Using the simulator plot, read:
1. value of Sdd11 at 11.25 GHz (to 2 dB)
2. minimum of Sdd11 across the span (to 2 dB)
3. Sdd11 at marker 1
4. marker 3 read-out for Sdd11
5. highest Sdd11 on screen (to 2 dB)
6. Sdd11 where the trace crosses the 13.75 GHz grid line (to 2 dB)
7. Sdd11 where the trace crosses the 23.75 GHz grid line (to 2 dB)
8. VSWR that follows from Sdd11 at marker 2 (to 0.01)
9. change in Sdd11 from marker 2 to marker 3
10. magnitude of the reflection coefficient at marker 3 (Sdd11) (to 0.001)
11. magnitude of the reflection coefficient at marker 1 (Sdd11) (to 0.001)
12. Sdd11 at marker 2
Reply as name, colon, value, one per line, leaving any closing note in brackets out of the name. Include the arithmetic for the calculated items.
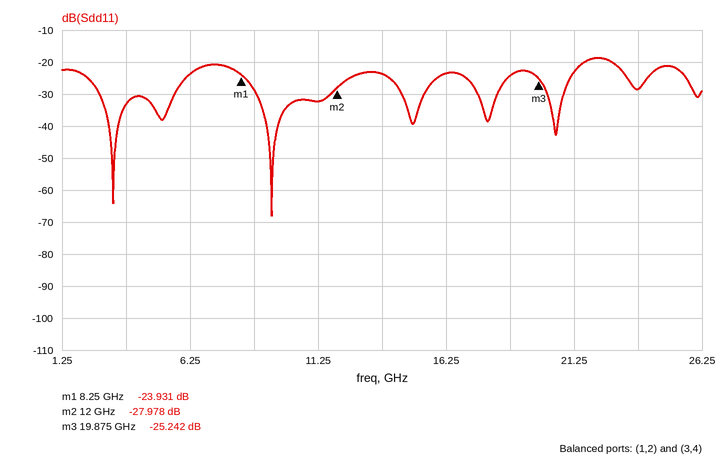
value of Sdd11 at 11.25 GHz: -32 dB
minimum of Sdd11 across the span: -68 dB
Sdd11 at marker 1: -23.931 dB
marker 3 read-out for Sdd11: -25.242 dB
highest Sdd11 on screen: -18 dB
Sdd11 where the trace crosses the 13.75 GHz grid line: -24 dB
Sdd11 where the trace crosses the 23.75 GHz grid line: -28 dB
VSWR that follows from Sdd11 at marker 2: (1 + 0.0399)/(1 − 0.0399) ≈ 1.08
change in Sdd11 from marker 2 to marker 3: -25.242 − (-27.978) = 2.736 dB
magnitude of the reflection coefficient at marker 3 (Sdd11): 10^(-25.242/20) ≈ 0.055
magnitude of the reflection coefficient at marker 1 (Sdd11): 10^(-23.931/20) ≈ 0.064
Sdd11 at marker 2: -27.978 dB
